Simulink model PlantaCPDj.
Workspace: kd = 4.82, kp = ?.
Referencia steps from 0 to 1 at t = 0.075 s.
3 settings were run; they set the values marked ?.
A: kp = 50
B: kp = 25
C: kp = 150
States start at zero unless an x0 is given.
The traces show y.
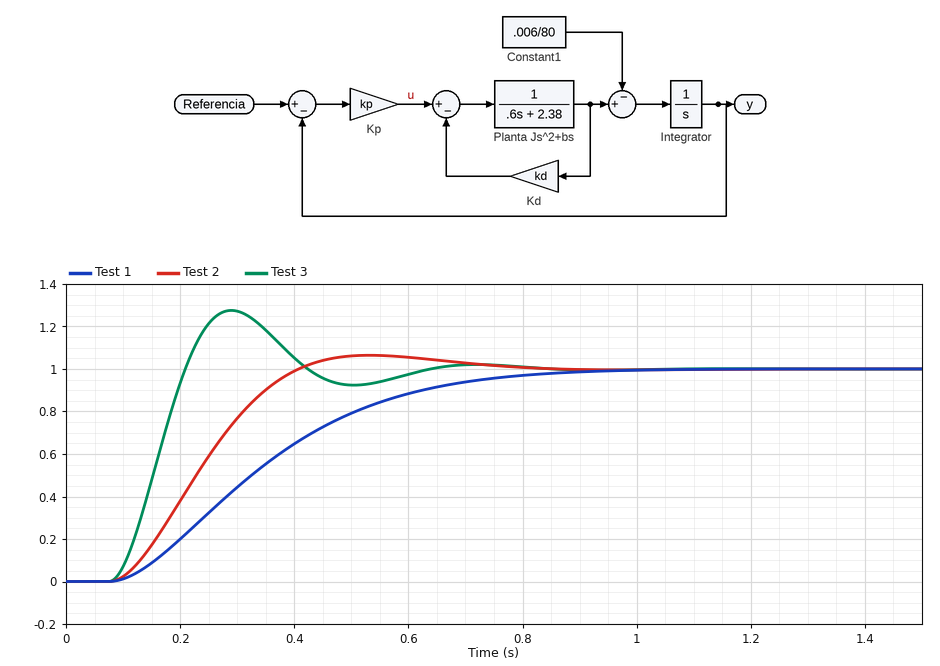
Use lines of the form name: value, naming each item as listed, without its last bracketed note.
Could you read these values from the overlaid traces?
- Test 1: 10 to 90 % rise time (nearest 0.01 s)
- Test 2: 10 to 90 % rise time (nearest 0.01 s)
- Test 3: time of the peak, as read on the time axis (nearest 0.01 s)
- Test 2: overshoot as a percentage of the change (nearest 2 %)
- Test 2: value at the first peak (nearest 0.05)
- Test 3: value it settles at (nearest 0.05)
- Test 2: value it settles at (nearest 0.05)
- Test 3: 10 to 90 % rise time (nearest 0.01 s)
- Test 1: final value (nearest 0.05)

Test 1: 10 to 90 % rise time: 0.47 s
Test 2: 10 to 90 % rise time: 0.22 s
Test 3: time of the peak, as read on the time axis: 0.29 s
Test 2: overshoot as a percentage of the change: 6 %
Test 2: value at the first peak: 1.05
Test 3: value it settles at: 1.00
Test 2: value it settles at: 1.00
Test 3: 10 to 90 % rise time: 0.09 s
Test 1: final value: 1.00
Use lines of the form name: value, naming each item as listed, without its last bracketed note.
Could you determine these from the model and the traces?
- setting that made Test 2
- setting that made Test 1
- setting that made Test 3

setting that made Test 2: A
setting that made Test 1: B
setting that made Test 3: C
